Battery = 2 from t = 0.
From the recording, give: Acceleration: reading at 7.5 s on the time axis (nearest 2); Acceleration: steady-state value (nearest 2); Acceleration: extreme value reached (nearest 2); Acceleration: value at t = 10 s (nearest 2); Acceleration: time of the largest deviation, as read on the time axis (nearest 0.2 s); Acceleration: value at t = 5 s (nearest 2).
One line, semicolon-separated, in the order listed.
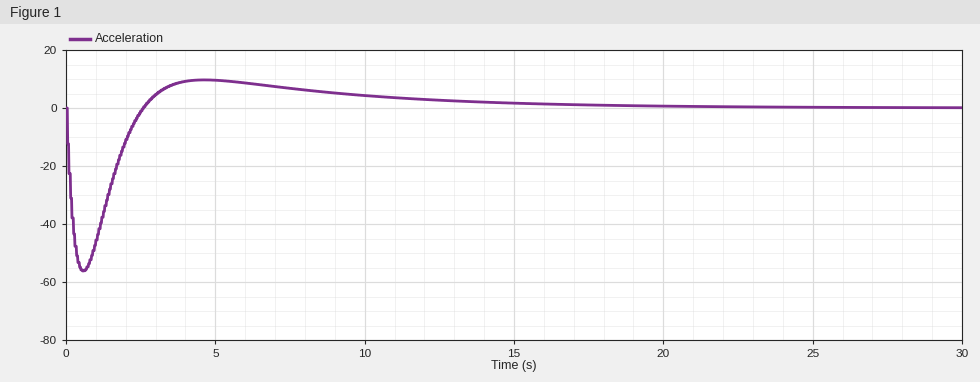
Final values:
6; 0; -56; 4; 0.6 s; 10
